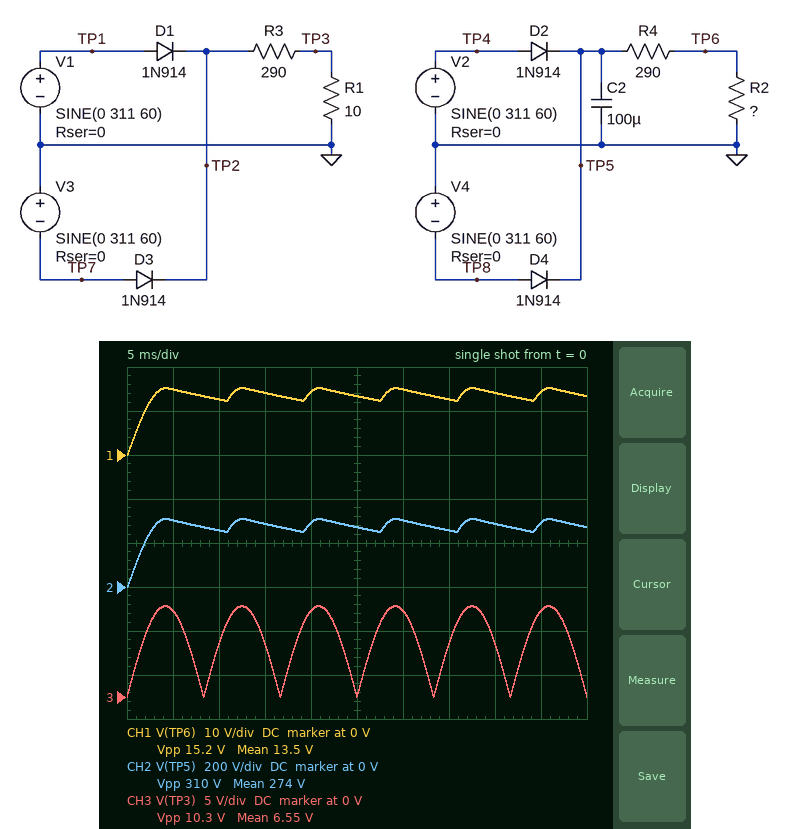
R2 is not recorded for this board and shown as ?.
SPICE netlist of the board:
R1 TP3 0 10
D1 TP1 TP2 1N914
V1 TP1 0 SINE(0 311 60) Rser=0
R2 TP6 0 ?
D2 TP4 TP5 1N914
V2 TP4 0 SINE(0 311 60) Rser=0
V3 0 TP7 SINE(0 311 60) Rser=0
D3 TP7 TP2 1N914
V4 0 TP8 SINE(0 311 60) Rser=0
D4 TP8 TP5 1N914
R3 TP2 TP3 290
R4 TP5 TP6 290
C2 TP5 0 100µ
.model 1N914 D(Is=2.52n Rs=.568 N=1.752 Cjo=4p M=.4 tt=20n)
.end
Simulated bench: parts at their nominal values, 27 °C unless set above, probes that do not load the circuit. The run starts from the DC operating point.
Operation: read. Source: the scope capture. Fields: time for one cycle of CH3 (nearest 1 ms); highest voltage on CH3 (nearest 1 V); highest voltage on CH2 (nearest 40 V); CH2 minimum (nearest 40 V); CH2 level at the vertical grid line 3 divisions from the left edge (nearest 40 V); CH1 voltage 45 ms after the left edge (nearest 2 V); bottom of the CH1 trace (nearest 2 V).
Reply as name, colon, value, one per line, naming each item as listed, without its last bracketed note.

time for one cycle of CH3: 8 ms
highest voltage on CH3: 10 V
highest voltage on CH2: 320 V
CH2 minimum: 0 V
CH2 level at the vertical grid line 3 divisions from the left edge: 280 V
CH1 voltage 45 ms after the left edge: 14 V
bottom of the CH1 trace: 0 V
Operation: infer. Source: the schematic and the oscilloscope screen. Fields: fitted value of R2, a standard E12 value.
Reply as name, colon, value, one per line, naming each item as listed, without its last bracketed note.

fitted value of R2, a standard E12 value: 15 Ω
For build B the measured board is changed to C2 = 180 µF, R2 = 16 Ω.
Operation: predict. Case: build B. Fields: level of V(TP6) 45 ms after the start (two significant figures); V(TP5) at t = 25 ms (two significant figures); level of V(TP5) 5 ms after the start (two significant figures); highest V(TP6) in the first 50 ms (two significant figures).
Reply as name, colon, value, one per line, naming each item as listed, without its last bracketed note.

level of V(TP6) 45 ms after the start: 15 V
V(TP5) at t = 25 ms: 290 V
level of V(TP5) 5 ms after the start: 310 V
highest V(TP6) in the first 50 ms: 16 V
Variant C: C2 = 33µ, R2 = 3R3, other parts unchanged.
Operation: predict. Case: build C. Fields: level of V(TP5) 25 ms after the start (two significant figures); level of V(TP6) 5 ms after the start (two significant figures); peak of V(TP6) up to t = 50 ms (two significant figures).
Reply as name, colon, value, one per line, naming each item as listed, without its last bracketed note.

level of V(TP5) 25 ms after the start: 210 V
level of V(TP6) 5 ms after the start: 3.3 V
peak of V(TP6) up to t = 50 ms: 3.5 V
